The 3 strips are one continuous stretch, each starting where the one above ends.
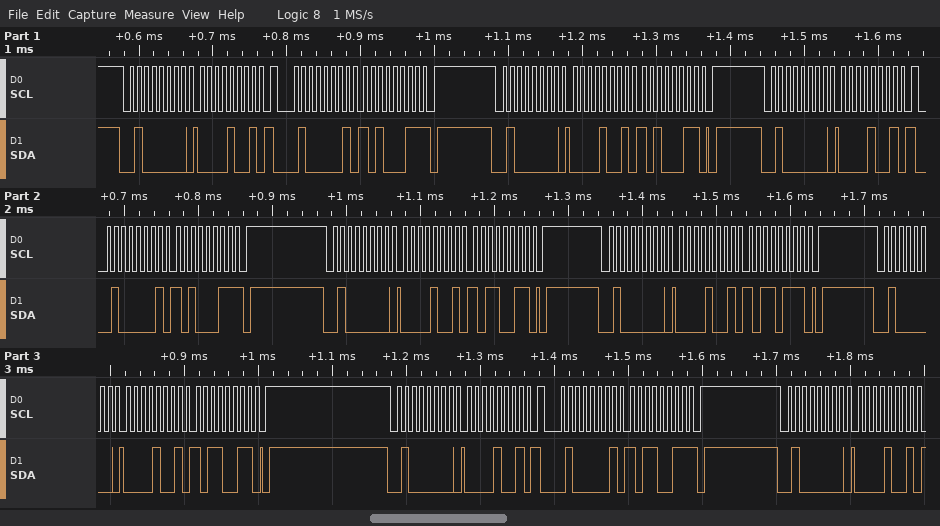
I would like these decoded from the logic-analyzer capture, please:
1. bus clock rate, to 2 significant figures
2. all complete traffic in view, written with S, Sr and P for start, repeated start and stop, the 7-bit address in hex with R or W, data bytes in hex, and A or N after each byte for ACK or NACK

100 kHz
S 20W A 09 A Sr 20R A A3 N P S 20W A 09 A A3 A P S 20W A 09 A Sr 20R A A3 N P S 20W A 09 A B3 A P S 20W A 09 A B7 A P S 20W A 09 A B3 A P S 20W A 09 A Sr 20R A B3 N P S 20W A 09 A
